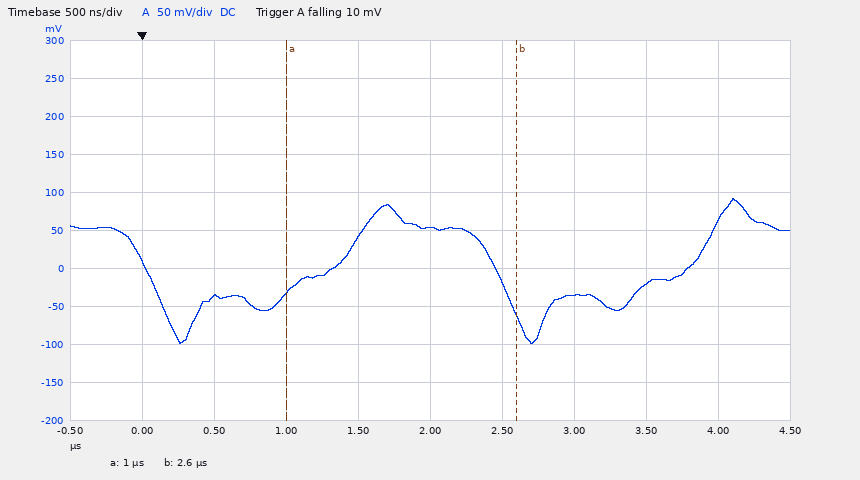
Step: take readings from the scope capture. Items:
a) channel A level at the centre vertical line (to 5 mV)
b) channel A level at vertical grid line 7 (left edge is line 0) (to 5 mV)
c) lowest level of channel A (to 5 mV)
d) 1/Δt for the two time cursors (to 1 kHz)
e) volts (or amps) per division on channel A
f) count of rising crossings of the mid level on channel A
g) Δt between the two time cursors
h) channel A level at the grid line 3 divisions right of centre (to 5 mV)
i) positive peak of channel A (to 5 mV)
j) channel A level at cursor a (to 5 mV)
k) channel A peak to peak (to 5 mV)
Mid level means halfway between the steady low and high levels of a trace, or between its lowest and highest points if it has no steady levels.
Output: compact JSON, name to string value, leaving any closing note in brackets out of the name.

{"channel A level at the centre vertical line": "55 mV", "channel A level at vertical grid line 7 (left edge is line 0)": "-35 mV", "lowest level of channel A": "-100 mV", "1/Δt for the two time cursors": "625 kHz", "volts (or amps) per division on channel A": "50 mV", "count of rising crossings of the mid level on channel A": "2", "Δt between the two time cursors": "1.60 µs", "channel A level at the grid line 3 divisions right of centre": "-20 mV", "positive peak of channel A": "90 mV", "channel A level at cursor a": "-30 mV", "channel A peak to peak": "190 mV"}
